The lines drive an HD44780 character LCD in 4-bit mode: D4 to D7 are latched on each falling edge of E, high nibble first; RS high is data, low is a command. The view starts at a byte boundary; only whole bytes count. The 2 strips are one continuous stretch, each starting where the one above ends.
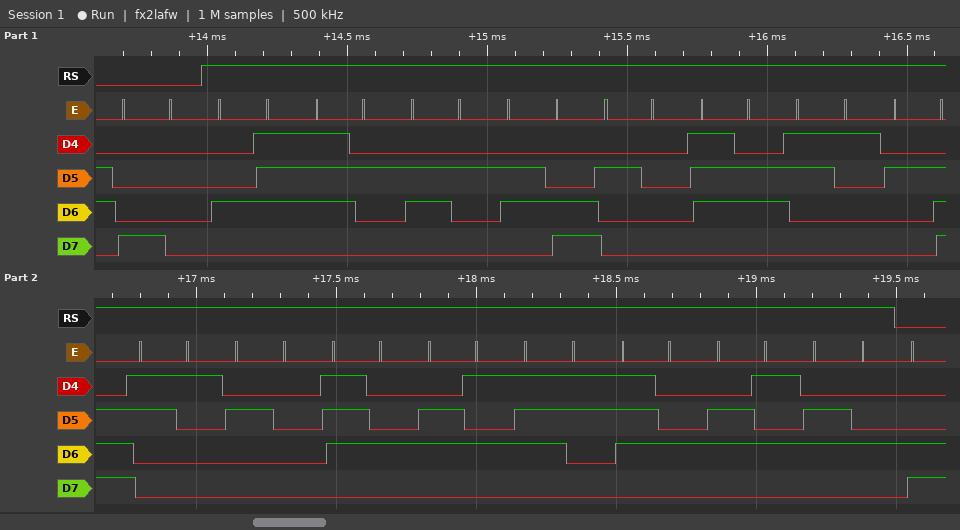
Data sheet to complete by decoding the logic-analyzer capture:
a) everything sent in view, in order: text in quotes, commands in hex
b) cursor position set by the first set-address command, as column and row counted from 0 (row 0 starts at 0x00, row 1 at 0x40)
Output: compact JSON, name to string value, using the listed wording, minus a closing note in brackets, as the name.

{"everything sent in view, in order: text in quotes, commands in hex": "0x80 \"Grbl v1.1 tested\"", "cursor position set by the first set-address command, as column and row counted from 0": "column 0, row 0"}
